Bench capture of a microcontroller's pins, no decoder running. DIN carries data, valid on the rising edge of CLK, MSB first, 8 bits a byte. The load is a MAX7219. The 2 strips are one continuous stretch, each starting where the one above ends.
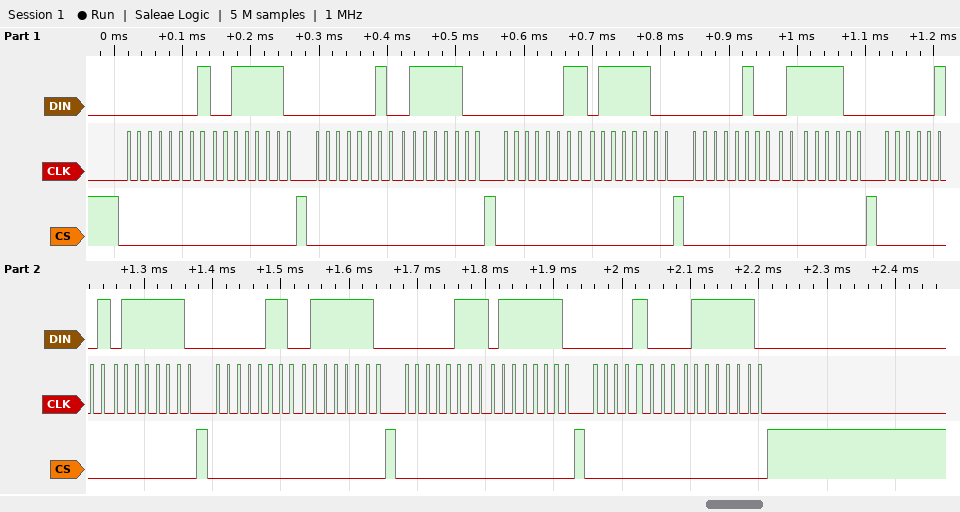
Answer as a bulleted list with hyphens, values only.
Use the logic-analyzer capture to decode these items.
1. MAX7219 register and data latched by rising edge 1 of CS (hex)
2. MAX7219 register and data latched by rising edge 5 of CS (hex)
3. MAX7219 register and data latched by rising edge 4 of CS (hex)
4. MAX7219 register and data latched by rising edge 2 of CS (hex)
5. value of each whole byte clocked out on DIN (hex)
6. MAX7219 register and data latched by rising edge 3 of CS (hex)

- register 0x1, data 0x3E
- register 0x5, data 0x7E
- register 0x4, data 0x7C
- register 0x2, data 0x7C
- 01 3E 02 7C 03 7C 04 7C 05 7E 06 7E 07 7E 08 7E
- register 0x3, data 0x7C
